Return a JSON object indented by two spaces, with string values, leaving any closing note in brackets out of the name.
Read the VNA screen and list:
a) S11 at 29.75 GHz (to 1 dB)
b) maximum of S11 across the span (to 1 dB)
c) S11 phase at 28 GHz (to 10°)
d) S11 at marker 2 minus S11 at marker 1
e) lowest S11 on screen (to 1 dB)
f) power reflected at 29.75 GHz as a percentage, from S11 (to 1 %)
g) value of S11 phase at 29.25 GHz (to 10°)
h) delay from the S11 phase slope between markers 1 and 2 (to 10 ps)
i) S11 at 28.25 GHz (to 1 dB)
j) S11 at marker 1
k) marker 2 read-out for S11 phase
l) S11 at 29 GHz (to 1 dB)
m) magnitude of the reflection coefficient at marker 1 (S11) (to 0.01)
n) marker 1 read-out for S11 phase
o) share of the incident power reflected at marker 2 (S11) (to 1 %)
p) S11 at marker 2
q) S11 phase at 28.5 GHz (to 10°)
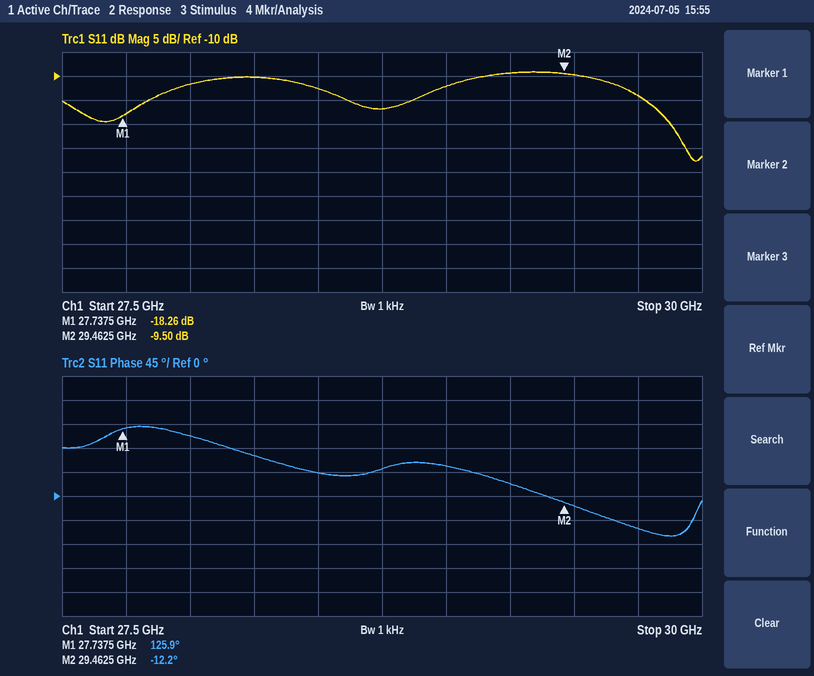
{
  "S11 at 29.75 GHz": "-14 dB",
  "maximum of S11 across the span": "-9 dB",
  "S11 phase at 28 GHz": "110°",
  "S11 at marker 2 minus S11 at marker 1": "8.76 dB",
  "lowest S11 on screen": "-28 dB",
  "power reflected at 29.75 GHz as a percentage, from S11": "4 %",
  "value of S11 phase at 29.25 GHz": "20°",
  "delay from the S11 phase slope between markers 1 and 2": "220 ps",
  "S11 at 28.25 GHz": "-10 dB",
  "S11 at marker 1": "-18.26 dB",
  "marker 2 read-out for S11 phase": "-12.2°",
  "S11 at 29 GHz": "-12 dB",
  "magnitude of the reflection coefficient at marker 1 (S11)": "0.12",
  "marker 1 read-out for S11 phase": "125.9°",
  "share of the incident power reflected at marker 2 (S11)": "11 %",
  "S11 at marker 2": "-9.50 dB",
  "S11 phase at 28.5 GHz": "40°"
}
